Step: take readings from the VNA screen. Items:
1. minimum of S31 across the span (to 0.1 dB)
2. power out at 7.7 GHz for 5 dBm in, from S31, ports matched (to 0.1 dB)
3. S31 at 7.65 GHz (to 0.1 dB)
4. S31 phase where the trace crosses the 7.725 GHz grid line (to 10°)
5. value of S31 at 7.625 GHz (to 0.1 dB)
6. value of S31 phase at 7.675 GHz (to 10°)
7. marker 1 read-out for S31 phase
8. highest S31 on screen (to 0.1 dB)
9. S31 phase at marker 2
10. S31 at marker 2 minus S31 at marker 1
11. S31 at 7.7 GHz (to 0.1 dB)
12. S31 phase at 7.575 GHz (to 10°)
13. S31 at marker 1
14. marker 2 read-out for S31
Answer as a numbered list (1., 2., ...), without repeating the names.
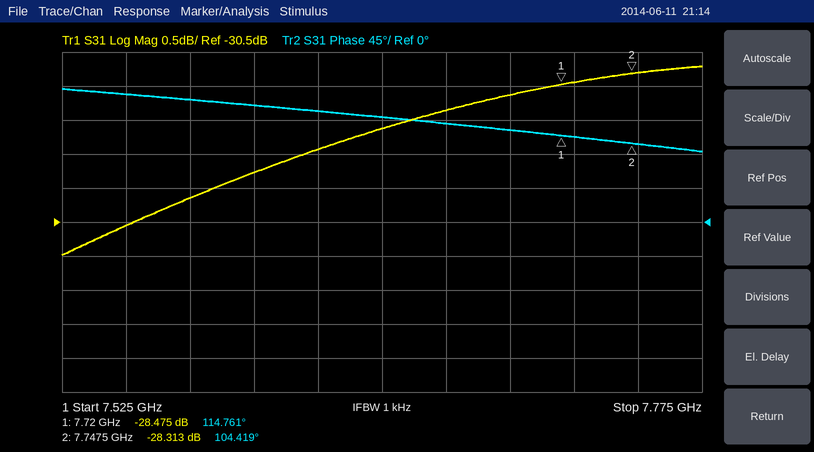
1. -31.0 dB
2. -23.6 dBm
3. -29.1 dB
4. 110°
5. -29.4 dB
6. 130°
7. 114.761°
8. -28.2 dB
9. 104.419°
10. 0.162 dB
11. -28.6 dB
12. 160°
13. -28.475 dB
14. -28.313 dB
